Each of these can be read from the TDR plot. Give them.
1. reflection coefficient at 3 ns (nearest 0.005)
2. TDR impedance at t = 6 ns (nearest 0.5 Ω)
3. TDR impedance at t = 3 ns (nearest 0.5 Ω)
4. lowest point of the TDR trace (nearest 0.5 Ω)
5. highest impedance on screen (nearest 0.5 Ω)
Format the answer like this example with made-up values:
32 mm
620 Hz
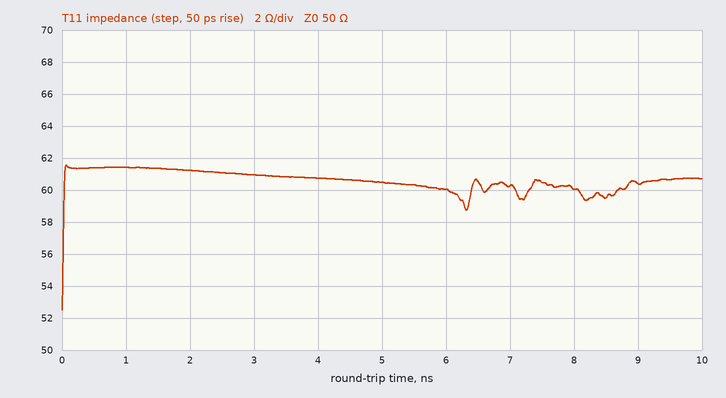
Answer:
+0.100
60.0 Ω
61.0 Ω
52.5 Ω
61.5 Ω
